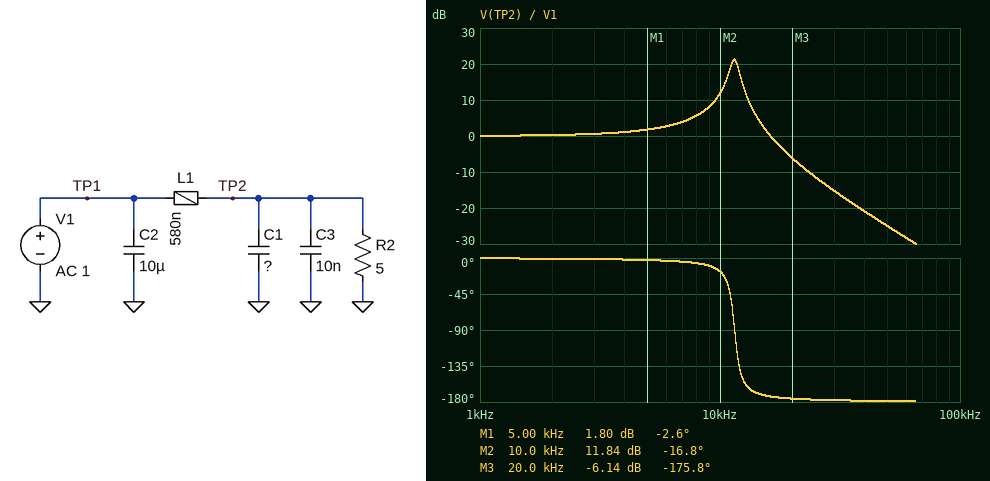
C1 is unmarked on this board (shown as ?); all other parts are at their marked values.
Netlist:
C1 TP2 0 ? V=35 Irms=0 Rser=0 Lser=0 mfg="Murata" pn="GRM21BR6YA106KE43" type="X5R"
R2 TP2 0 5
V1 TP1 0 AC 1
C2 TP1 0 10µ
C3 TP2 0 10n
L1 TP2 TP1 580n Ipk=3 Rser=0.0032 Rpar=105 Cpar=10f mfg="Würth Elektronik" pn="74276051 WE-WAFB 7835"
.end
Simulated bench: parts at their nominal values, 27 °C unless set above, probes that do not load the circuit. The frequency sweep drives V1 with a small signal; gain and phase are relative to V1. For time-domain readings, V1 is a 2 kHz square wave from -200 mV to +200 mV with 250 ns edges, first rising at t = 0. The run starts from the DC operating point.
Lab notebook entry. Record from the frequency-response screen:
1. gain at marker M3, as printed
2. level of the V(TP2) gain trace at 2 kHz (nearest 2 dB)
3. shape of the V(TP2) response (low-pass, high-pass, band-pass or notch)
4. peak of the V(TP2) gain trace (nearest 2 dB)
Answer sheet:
-6.14 dB
0 dB
low-pass
22 dB
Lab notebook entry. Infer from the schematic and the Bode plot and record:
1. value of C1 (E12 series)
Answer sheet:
330 µF
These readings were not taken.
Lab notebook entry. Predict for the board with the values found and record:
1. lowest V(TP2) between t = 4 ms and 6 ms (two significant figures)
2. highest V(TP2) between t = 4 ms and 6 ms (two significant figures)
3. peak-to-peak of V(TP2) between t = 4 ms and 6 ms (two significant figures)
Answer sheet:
-460 mV
460 mV
920 mV
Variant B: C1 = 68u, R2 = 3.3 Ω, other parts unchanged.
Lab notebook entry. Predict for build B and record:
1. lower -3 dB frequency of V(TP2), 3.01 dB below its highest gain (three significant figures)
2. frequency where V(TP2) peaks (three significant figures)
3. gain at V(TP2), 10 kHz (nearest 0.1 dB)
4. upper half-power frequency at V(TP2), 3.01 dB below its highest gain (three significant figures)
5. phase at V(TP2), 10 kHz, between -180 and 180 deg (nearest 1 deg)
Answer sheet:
24.5 kHz
25.3 kHz
1.5 dB
26.1 kHz
-2 deg
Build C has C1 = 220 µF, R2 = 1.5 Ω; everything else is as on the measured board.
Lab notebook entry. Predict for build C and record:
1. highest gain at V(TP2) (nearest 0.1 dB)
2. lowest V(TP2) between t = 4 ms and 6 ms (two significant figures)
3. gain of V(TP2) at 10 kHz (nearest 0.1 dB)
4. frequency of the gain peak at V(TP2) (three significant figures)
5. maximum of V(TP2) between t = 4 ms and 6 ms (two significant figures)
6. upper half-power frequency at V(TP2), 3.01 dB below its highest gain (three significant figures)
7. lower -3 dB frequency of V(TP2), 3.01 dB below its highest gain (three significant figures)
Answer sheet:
20.3 dB
-720 mV
6.0 dB
14.1 kHz
720 mV
14.7 kHz
13.4 kHz
